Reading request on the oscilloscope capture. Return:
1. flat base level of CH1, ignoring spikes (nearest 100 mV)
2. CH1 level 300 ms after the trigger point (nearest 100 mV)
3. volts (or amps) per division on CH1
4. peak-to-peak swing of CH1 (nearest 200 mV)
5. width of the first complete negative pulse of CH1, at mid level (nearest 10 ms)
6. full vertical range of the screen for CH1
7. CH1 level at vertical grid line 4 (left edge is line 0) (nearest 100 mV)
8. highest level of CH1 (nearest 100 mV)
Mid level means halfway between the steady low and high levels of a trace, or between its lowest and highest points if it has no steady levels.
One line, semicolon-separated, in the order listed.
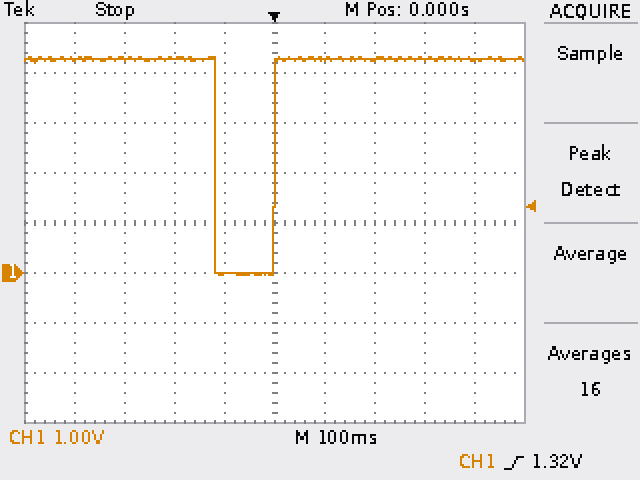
0.0 V; 4.3 V; 1 V; 4.4 V; 120 ms; 8 V; 0.0 V; 4.3 V
